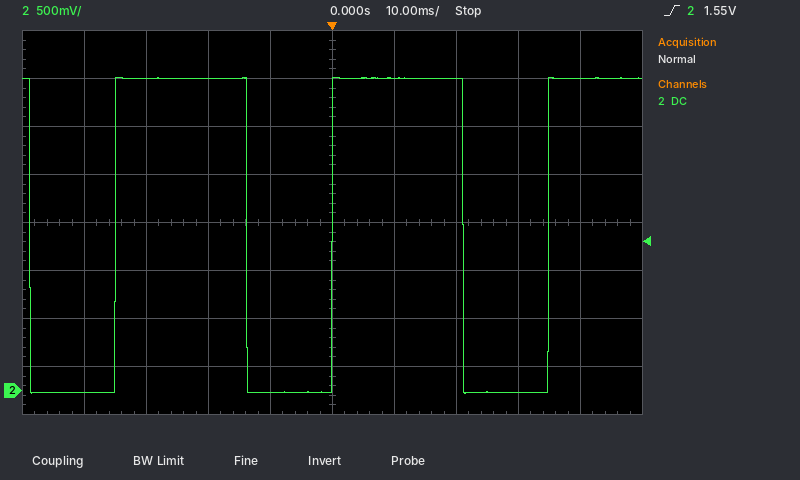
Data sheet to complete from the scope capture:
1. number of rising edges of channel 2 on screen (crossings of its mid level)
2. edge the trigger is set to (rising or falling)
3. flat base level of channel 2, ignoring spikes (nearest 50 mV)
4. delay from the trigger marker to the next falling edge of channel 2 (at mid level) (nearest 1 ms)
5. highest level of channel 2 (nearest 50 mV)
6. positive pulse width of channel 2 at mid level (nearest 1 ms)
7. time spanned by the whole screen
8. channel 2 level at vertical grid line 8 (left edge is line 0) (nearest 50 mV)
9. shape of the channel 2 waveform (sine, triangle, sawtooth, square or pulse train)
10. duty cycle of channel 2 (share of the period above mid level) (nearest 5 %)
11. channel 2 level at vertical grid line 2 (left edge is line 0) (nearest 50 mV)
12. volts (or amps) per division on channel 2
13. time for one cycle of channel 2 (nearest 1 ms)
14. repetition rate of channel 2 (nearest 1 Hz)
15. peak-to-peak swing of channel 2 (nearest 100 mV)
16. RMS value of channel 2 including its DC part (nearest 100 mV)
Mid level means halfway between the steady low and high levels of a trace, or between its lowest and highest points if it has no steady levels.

3
rising
0 mV
21 ms
3.25 V
21 ms
100 ms
0 mV
pulse train
60 %
3.25 V
500 mV
35 ms
29 Hz
3.30 V
2.5 V
